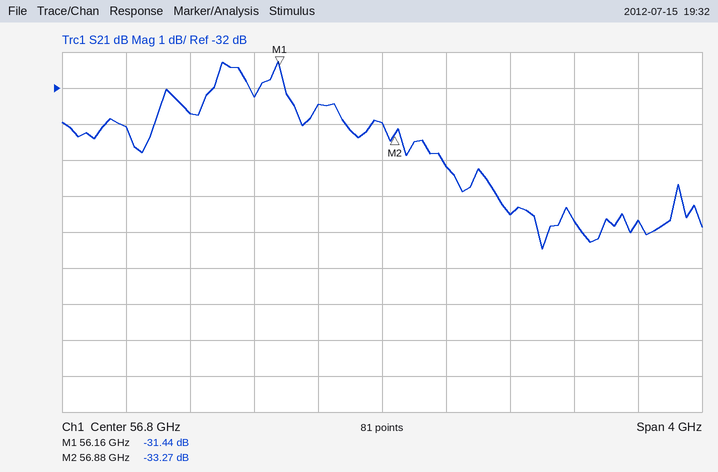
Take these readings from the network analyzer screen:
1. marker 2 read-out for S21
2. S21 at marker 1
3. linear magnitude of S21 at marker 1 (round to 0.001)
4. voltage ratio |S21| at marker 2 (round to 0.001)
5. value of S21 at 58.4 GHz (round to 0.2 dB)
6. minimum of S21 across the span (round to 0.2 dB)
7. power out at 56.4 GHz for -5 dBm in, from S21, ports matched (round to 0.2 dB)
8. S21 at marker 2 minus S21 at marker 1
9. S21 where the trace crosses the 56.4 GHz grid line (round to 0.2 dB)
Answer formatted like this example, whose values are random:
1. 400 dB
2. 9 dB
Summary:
1. -33.27 dB
2. -31.44 dB
3. 0.027
4. 0.022
5. -35.6 dB
6. -36.4 dB
7. -37.4 dBm
8. -1.83 dB
9. -32.4 dB
